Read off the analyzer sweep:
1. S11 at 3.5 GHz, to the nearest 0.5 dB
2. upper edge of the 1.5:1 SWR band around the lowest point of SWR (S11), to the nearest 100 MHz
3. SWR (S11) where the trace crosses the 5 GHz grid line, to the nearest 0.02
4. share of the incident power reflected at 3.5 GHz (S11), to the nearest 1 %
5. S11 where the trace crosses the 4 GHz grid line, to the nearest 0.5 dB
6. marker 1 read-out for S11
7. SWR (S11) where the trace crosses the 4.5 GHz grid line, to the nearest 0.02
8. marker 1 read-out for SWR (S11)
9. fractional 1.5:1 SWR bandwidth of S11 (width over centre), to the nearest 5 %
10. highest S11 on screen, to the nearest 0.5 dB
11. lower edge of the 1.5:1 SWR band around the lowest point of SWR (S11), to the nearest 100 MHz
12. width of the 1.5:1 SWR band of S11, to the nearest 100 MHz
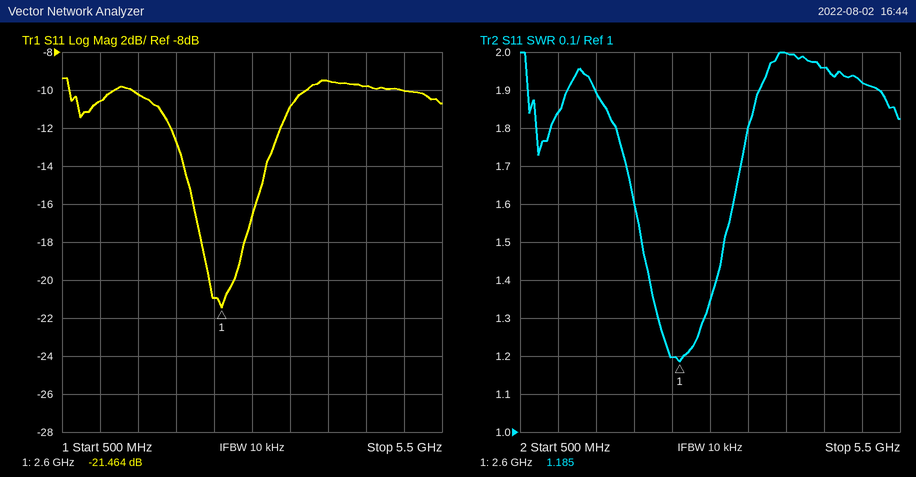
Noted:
-11.0 dB
3.2 GHz
1.92
8 %
-9.5 dB
-21.464 dB
1.96
1.185
40 %
-9.5 dB
2.1 GHz
1.1 GHz
